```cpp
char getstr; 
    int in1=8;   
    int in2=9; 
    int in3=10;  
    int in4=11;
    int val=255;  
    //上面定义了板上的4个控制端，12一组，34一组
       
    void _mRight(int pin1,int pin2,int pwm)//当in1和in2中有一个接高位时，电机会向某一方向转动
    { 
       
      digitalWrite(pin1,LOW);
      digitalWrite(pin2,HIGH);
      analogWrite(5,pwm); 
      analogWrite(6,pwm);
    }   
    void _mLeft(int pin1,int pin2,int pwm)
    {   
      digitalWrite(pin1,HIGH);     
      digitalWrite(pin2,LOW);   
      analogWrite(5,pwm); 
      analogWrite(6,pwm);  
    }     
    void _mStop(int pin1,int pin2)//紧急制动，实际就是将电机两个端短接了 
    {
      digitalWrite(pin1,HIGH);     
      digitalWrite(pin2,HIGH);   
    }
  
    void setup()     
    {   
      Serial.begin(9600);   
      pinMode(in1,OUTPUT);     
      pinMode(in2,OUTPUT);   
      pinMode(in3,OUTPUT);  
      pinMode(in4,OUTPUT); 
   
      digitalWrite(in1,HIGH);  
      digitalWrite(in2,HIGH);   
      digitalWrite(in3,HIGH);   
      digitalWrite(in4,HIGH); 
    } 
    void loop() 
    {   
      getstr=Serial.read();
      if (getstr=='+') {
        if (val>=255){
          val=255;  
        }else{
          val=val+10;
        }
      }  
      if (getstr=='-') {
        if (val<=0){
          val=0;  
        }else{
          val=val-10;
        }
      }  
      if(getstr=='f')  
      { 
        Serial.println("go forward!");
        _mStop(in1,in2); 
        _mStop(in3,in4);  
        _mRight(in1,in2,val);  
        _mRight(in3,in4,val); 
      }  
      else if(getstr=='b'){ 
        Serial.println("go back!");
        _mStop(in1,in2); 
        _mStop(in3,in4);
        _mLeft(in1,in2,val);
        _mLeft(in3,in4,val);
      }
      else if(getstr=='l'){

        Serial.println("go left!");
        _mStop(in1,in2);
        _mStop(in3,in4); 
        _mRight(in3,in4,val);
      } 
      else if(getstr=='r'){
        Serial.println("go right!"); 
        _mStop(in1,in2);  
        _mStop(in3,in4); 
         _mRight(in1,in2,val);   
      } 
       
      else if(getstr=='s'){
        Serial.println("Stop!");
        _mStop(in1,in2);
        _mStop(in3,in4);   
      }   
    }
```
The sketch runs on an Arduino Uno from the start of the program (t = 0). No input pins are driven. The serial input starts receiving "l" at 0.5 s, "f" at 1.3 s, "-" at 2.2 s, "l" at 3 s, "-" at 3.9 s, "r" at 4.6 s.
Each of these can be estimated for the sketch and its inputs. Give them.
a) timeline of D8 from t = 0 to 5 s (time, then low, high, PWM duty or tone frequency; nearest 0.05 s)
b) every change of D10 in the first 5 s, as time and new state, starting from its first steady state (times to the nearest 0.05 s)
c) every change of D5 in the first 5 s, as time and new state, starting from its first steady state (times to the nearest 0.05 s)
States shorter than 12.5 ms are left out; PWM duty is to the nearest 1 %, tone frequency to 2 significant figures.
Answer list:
0 s high; 1.3 s low; 3 s high; 4.6 s low
0 s high; 0.5 s low; 4.6 s high
0.5 s high; 3 s PWM 96 %; 4.6 s PWM 92 %
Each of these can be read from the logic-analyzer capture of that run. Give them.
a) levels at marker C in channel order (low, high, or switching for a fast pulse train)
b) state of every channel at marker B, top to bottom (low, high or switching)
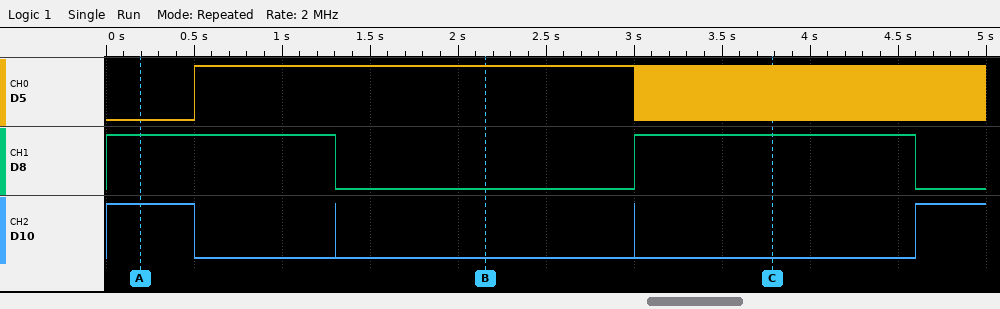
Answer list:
D5 switching, D8 high, D10 low
D5 high, D8 low, D10 low
